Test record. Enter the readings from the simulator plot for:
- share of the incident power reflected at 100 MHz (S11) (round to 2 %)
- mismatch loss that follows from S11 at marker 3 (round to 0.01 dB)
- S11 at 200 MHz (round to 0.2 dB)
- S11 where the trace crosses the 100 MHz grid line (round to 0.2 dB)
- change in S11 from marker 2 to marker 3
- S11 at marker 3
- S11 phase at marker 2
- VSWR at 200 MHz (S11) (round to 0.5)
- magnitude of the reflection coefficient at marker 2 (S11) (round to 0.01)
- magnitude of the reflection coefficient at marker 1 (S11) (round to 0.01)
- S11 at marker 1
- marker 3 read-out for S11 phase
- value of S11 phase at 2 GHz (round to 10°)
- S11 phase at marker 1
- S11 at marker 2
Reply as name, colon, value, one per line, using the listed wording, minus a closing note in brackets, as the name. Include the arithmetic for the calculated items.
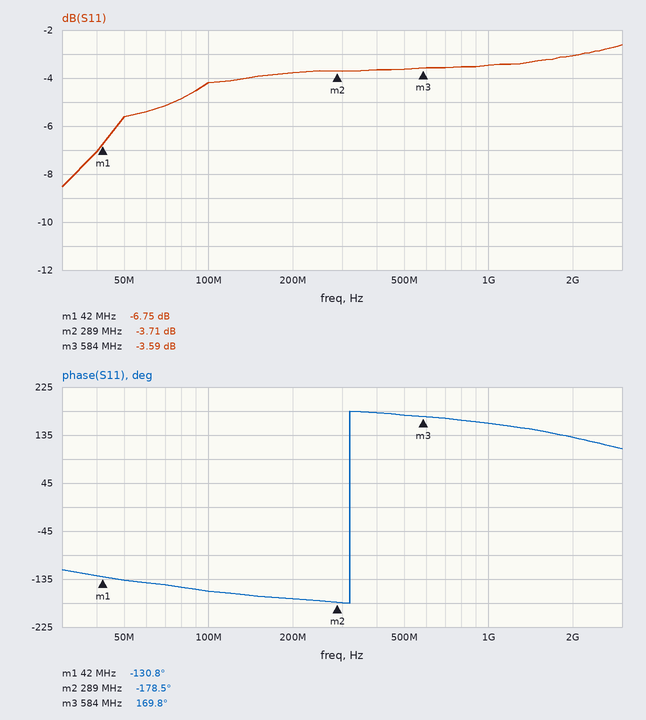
share of the incident power reflected at 100 MHz (S11): 10^(-4.2/10) ≈ 38 %
mismatch loss that follows from S11 at marker 3: −10 log10(1 − 10^(-3.59/10)) ≈ 2.50 dB
S11 at 200 MHz: -3.8 dB
S11 where the trace crosses the 100 MHz grid line: -4.2 dB
change in S11 from marker 2 to marker 3: -3.59 − (-3.71) = 0.12 dB
S11 at marker 3: -3.59 dB
S11 phase at marker 2: -178.5°
VSWR at 200 MHz (S11): |Γ| = 10^(-3.8/20) = 0.6457; VSWR = (1 + 0.6457)/(1 − 0.6457) ≈ 4.64, so 4.5 to the nearest 0.5
magnitude of the reflection coefficient at marker 2 (S11): 10^(-3.71/20) ≈ 0.65
magnitude of the reflection coefficient at marker 1 (S11): 10^(-6.75/20) ≈ 0.46
S11 at marker 1: -6.75 dB
marker 3 read-out for S11 phase: 169.8°
value of S11 phase at 2 GHz: 130°
S11 phase at marker 1: -130.8°
S11 at marker 2: -3.71 dB
